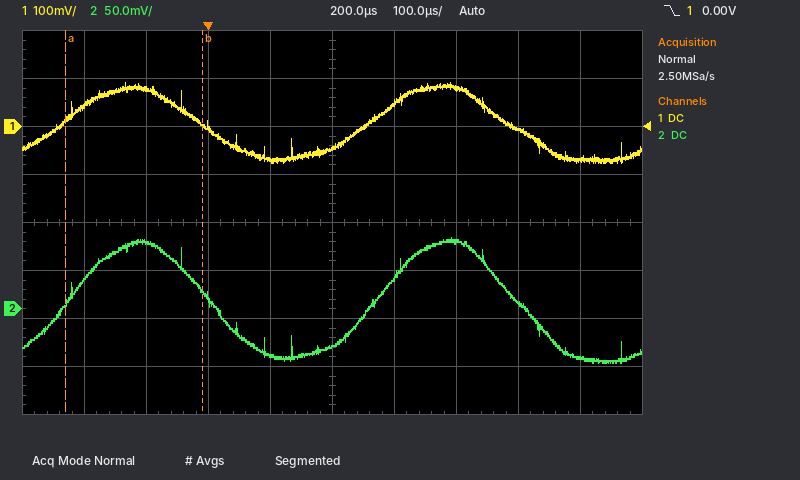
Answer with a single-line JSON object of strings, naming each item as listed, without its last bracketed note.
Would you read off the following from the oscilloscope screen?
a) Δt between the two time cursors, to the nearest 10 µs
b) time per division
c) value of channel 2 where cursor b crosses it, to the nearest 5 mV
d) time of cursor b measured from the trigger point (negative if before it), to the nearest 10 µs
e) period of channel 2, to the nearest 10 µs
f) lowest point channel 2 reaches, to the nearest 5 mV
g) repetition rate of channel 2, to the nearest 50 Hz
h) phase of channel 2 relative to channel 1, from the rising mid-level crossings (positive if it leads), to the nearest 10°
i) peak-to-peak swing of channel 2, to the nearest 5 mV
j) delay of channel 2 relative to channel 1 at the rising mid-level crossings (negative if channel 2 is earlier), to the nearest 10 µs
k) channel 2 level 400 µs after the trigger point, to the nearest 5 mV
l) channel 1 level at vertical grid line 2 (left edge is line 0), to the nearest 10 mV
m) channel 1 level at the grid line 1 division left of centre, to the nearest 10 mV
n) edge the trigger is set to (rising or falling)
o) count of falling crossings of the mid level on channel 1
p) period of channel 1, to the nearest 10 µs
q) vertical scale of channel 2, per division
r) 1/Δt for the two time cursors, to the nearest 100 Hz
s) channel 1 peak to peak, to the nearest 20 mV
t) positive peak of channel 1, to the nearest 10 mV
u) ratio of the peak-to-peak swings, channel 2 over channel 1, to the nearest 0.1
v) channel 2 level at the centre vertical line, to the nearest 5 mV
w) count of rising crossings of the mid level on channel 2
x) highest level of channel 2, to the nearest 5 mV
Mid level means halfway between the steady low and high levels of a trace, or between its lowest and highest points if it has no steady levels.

{"Δt between the two time cursors, to the nearest 10 µs": "220 µs", "time per division": "100 µs", "value of channel 2 where cursor b crosses it, to the nearest 5 mV": "20 mV", "time of cursor b measured from the trigger point (negative if before it), to the nearest 10 µs": "-10 µs", "period of channel 2, to the nearest 10 µs": "500 µs", "lowest point channel 2 reaches, to the nearest 5 mV": "-55 mV", "repetition rate of channel 2, to the nearest 50 Hz": "2.00 kHz", "phase of channel 2 relative to channel 1, from the rising mid-level crossings (positive if it leads), to the nearest 10°": "-10°", "peak-to-peak swing of channel 2, to the nearest 5 mV": "130 mV", "delay of channel 2 relative to channel 1 at the rising mid-level crossings (negative if channel 2 is earlier), to the nearest 10 µs": "+10 µs", "channel 2 level 400 µs after the trigger point, to the nearest 5 mV": "70 mV", "channel 1 level at vertical grid line 2 (left edge is line 0), to the nearest 10 mV": "80 mV", "channel 1 level at the grid line 1 division left of centre, to the nearest 10 mV": "-70 mV", "edge the trigger is set to": "falling", "count of falling crossings of the mid level on channel 1": "2", "period of channel 1, to the nearest 10 µs": "490 µs", "vertical scale of channel 2, per division": "50 mV", "1/Δt for the two time cursors, to the nearest 100 Hz": "4.5 kHz", "channel 1 peak to peak, to the nearest 20 mV": "160 mV", "positive peak of channel 1, to the nearest 10 mV": "90 mV", "ratio of the peak-to-peak swings, channel 2 over channel 1, to the nearest 0.1": "0.8", "channel 2 level at the centre vertical line, to the nearest 5 mV": "-40 mV", "count of rising crossings of the mid level on channel 2": "2", "highest level of channel 2, to the nearest 5 mV": "75 mV"}
